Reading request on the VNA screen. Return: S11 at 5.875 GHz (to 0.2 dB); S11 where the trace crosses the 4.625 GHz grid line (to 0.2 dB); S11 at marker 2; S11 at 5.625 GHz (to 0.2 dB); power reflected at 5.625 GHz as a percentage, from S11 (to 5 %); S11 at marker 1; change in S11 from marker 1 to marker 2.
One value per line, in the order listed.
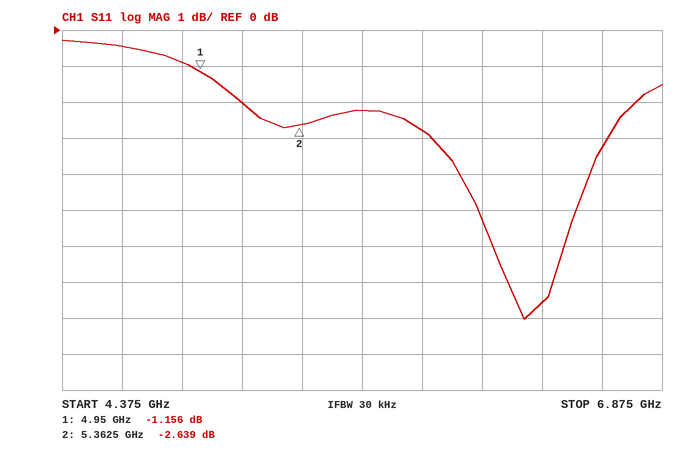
-2.8 dB
-0.4 dB
-2.639 dB
-2.2 dB
60 %
-1.156 dB
-1.483 dB
